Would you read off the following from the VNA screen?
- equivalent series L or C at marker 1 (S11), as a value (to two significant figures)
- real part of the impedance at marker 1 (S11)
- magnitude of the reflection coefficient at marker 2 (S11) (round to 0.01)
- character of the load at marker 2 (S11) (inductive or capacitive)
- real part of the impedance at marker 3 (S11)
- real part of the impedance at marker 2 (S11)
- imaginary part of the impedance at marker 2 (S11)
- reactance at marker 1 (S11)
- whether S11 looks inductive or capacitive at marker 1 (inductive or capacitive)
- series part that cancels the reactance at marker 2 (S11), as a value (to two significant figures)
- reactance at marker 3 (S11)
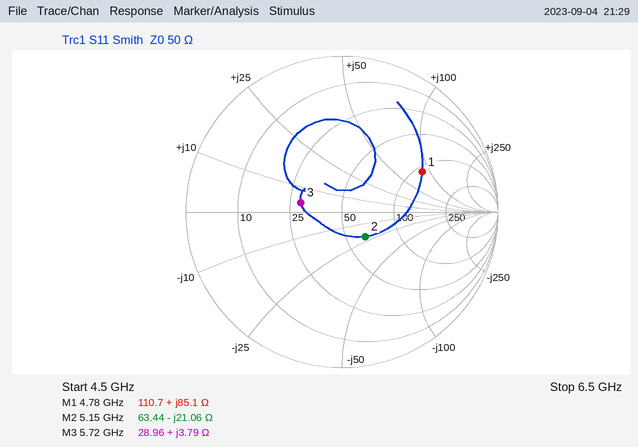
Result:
2.8 nH
110.7 Ω
0.22
capacitive
28.96 Ω
63.44 Ω
-21.06 Ω
+85.1 Ω
inductive
650 pH
+3.79 Ω
